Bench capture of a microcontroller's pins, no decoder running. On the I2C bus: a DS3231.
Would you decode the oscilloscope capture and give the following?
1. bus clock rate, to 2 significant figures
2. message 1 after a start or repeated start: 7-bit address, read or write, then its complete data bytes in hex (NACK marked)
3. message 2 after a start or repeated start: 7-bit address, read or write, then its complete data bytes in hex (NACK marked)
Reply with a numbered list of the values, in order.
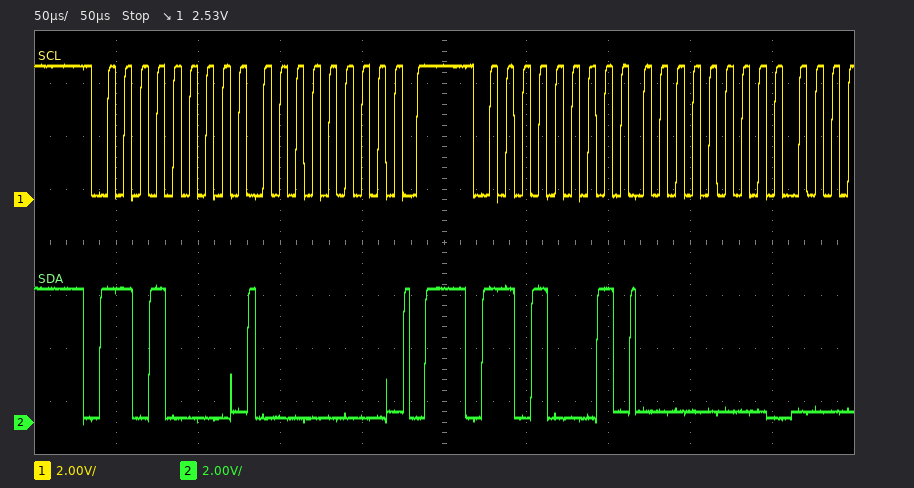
1. 100 kHz
2. 0x68 write: 00
3. 0x68 read: 00
